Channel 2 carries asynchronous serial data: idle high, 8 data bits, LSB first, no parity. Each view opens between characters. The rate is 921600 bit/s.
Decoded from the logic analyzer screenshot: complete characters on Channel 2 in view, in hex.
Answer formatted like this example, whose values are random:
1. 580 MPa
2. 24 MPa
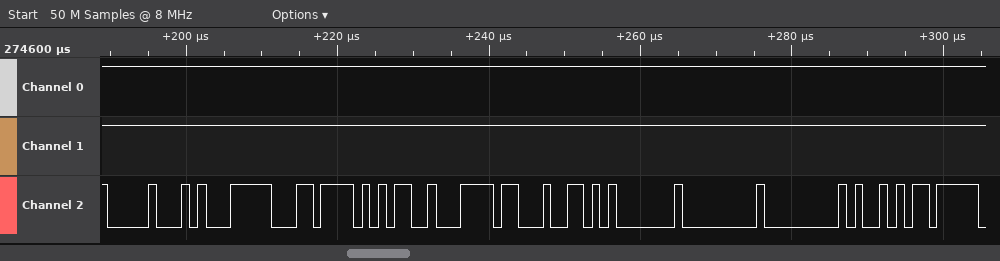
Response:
1. 10, F1, EC, 35, BC, 64, 01, 00, 00, A9
